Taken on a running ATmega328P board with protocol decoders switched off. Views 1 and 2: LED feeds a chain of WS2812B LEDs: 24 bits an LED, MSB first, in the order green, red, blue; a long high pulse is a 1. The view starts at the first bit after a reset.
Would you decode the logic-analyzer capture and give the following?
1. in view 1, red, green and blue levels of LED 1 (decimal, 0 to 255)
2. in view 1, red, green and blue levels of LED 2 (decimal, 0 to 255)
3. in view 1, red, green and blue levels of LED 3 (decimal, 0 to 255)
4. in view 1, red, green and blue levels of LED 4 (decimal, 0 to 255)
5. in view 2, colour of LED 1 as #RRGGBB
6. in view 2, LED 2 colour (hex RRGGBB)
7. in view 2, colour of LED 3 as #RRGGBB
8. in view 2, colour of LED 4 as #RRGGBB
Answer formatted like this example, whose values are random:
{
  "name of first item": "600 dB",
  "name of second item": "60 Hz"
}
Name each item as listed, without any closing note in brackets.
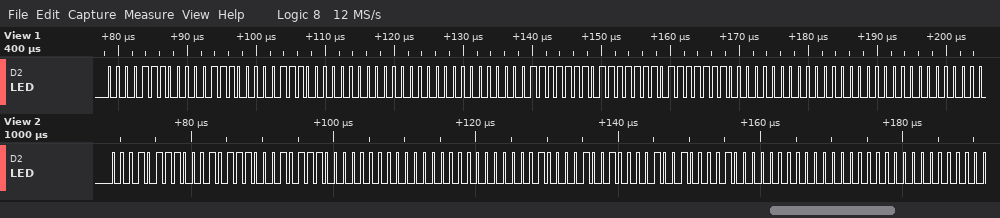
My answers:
{
  "in view 1, red, green and blue levels of LED 1": "14, 14, 14",
  "in view 1, red, green and blue levels of LED 2": "0, 0, 0",
  "in view 1, red, green and blue levels of LED 3": "127, 127, 127",
  "in view 1, red, green and blue levels of LED 4": "0, 0, 0",
  "in view 2, colour of LED 1 as #RRGGBB": "#171717",
  "in view 2, LED 2 colour": "#000000",
  "in view 2, colour of LED 3 as #RRGGBB": "#848484",
  "in view 2, colour of LED 4 as #RRGGBB": "#000000"
}
